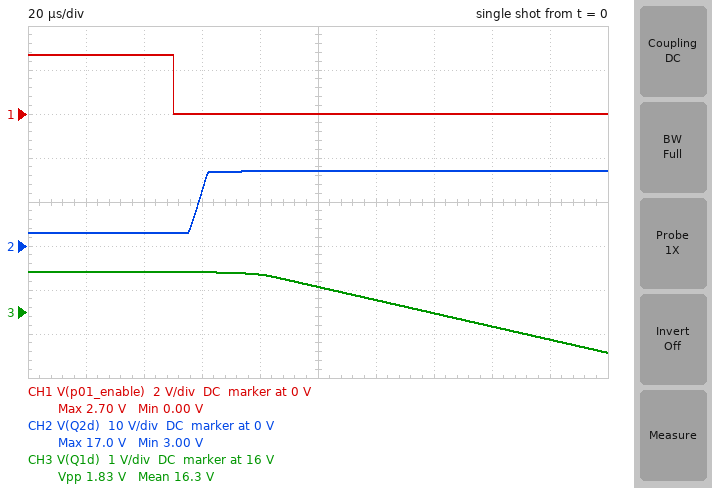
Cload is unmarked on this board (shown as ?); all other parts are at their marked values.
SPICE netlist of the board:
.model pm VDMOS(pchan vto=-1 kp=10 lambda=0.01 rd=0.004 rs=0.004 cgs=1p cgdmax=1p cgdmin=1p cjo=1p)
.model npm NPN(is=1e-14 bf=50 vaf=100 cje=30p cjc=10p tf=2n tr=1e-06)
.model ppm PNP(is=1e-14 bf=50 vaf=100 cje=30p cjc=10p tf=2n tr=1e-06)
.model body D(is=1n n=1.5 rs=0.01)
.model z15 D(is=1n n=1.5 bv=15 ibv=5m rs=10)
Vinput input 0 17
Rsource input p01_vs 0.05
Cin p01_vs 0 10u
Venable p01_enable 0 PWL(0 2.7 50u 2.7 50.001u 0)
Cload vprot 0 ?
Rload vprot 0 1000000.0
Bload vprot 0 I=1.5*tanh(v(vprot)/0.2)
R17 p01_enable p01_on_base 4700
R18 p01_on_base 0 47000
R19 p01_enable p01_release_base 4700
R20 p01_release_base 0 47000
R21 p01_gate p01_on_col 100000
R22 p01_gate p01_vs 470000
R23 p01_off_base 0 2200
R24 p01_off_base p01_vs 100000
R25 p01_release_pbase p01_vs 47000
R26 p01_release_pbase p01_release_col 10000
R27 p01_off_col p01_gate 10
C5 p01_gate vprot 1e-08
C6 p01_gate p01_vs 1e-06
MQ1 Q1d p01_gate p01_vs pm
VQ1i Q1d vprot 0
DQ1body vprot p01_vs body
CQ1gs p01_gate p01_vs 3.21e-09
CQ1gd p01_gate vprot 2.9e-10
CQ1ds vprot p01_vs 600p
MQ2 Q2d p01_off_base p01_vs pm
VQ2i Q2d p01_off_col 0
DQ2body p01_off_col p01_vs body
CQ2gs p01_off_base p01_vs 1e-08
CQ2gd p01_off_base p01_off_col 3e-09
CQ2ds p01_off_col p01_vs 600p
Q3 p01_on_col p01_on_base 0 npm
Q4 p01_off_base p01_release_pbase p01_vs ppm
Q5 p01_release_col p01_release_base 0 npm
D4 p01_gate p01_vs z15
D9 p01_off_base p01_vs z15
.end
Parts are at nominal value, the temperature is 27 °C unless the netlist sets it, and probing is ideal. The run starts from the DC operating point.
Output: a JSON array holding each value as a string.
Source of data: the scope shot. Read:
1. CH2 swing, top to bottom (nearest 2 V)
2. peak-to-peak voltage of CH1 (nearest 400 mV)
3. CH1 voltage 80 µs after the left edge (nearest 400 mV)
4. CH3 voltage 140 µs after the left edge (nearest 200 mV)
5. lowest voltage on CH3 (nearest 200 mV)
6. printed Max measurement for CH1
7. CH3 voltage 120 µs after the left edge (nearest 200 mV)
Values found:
["14 V", "2.8 V", "0 V", "16.0 V", "15.0 V", "2.70 V", "16.2 V"]
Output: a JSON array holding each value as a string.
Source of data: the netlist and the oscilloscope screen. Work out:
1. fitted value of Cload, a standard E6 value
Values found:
["100 µF"]
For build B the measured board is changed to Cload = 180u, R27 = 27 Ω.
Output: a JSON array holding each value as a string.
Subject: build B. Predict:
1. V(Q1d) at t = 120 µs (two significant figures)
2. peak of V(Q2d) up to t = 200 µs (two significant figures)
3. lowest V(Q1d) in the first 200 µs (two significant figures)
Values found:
["17 V", "17 V", "16 V"]
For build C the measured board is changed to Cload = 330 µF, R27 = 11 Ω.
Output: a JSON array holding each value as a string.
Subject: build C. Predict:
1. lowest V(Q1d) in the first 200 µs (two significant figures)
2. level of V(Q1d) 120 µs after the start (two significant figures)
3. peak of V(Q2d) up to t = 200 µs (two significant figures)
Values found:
["16 V", "17 V", "17 V"]
